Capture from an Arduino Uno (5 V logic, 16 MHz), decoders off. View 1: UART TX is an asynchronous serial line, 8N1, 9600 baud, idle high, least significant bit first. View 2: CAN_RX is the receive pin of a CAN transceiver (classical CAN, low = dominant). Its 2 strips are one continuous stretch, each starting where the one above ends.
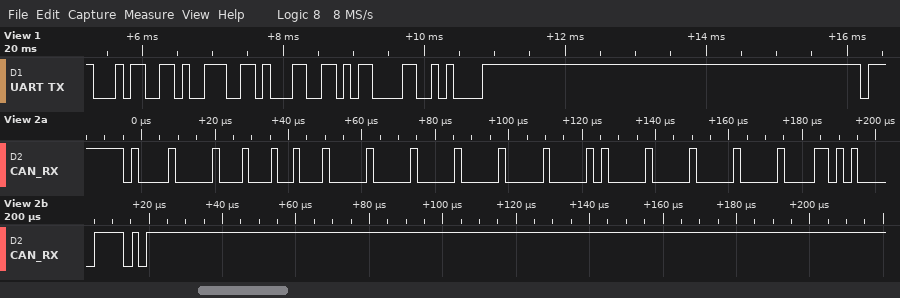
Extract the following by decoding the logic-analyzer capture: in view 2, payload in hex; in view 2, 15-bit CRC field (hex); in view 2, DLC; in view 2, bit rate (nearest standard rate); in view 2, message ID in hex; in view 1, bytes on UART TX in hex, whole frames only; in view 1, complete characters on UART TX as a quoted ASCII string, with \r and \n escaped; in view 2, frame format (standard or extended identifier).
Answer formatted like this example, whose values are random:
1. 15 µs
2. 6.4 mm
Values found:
1. 91 00 00 00 01 00 00 00
2. 0x6A0E
3. 8
4. 500 kbit/s
5. 0x420
6. 34 39 31 0D 0A
7. "491\r\n"
8. standard
